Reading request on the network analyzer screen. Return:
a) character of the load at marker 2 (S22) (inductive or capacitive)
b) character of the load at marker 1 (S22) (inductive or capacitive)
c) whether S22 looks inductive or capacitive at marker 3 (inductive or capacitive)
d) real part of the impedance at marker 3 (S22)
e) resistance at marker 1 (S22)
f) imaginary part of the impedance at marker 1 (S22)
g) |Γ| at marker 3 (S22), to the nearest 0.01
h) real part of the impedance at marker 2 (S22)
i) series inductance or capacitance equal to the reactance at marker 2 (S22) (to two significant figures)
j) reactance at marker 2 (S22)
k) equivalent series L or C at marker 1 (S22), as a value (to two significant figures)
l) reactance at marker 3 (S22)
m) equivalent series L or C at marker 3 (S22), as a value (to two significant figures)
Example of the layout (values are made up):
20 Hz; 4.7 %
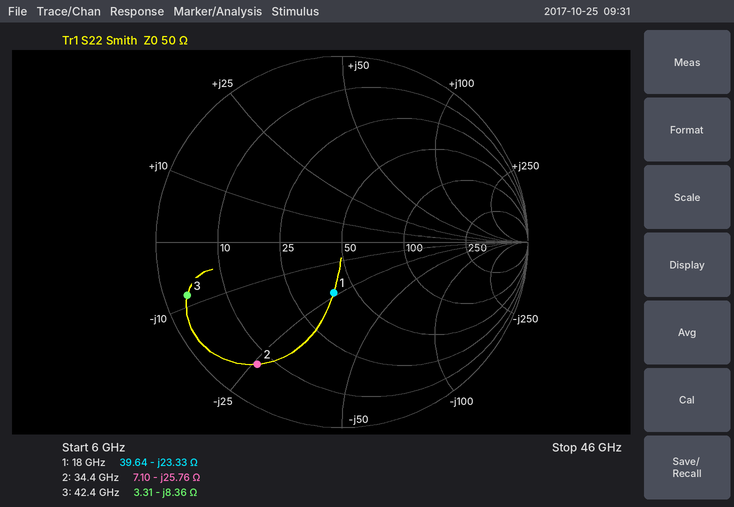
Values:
capacitive; capacitive; capacitive; 3.31 Ω; 39.64 Ω; -23.33 Ω; 0.88; 7.10 Ω; 180 fF; -25.76 Ω; 380 fF; -8.36 Ω; 450 fF
